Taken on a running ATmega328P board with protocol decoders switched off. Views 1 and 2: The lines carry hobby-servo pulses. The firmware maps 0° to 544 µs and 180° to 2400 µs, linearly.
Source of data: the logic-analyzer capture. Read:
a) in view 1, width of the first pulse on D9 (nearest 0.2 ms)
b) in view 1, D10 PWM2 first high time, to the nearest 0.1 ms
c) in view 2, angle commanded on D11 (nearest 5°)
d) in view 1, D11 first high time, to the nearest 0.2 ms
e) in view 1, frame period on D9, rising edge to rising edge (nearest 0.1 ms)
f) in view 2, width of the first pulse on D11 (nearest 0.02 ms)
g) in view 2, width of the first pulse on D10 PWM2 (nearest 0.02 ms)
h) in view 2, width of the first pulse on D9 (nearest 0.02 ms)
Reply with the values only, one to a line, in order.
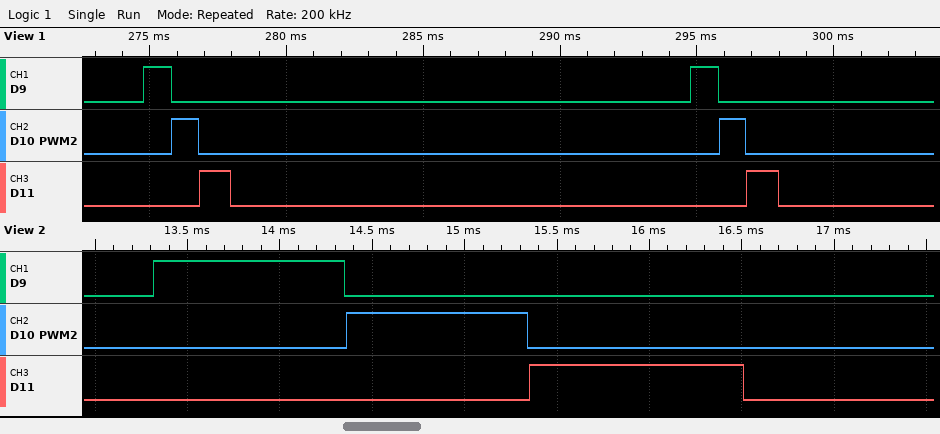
1.0 ms
1.0 ms
60°
1.2 ms
20.0 ms
1.16 ms
0.98 ms
1.04 ms
